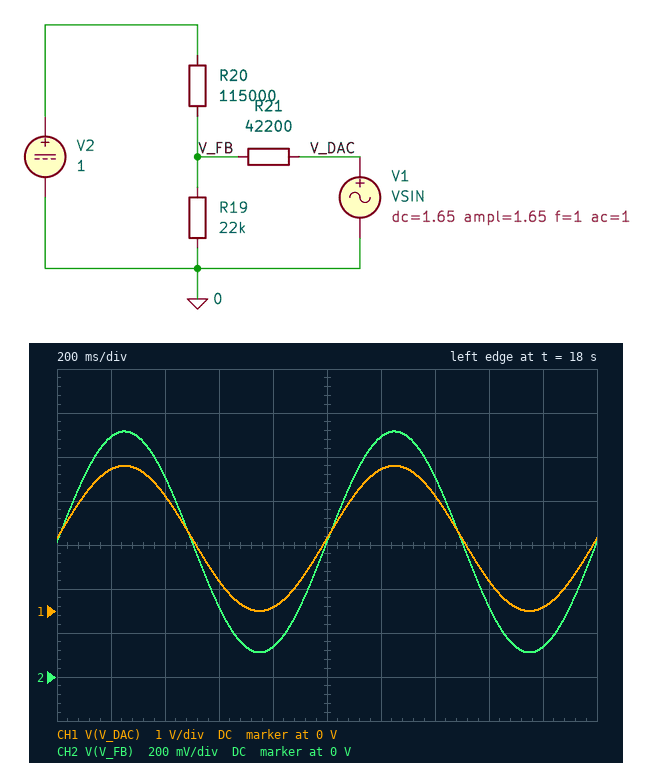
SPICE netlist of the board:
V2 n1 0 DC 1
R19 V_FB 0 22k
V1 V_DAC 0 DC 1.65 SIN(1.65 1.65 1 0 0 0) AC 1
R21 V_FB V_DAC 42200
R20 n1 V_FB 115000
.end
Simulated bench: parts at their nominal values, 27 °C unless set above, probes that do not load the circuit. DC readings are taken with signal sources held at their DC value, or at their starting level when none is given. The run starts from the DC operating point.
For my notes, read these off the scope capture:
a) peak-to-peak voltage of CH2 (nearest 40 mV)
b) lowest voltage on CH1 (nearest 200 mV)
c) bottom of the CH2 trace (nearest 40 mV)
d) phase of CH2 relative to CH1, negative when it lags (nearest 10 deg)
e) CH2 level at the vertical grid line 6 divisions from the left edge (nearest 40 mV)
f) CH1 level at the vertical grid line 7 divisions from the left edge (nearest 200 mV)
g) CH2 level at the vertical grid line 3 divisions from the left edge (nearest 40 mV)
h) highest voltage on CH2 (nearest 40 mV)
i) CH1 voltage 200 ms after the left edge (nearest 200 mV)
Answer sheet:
1.00 V
0 V
120 mV
0 deg
1.08 V
2.6 V
320 mV
1.12 V
3.2 V
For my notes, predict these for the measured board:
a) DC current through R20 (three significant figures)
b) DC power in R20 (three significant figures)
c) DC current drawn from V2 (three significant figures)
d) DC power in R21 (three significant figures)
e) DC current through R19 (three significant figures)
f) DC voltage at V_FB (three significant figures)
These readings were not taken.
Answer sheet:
3.36 µA
1.30 µW
3.36 µA
25.4 µW
27.9 µA
614 mV
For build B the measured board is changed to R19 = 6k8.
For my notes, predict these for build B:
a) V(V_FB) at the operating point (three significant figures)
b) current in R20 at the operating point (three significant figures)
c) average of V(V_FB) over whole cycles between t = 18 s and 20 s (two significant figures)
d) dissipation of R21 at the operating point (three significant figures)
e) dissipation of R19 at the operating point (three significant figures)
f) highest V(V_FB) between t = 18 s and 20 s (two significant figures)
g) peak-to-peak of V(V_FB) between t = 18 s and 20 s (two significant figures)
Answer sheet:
266 mV
6.38 µA
270 mV
45.4 µW
10.4 µW
480 mV
440 mV
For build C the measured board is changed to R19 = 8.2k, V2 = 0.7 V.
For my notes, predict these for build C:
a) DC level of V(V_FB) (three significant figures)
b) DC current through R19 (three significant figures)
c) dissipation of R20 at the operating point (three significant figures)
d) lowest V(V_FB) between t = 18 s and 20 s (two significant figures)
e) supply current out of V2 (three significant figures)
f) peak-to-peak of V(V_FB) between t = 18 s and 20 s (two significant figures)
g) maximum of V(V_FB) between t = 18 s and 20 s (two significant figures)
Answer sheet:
293 mV
35.7 µA
1.44 µW
39 mV
3.54 µA
510 mV
550 mV
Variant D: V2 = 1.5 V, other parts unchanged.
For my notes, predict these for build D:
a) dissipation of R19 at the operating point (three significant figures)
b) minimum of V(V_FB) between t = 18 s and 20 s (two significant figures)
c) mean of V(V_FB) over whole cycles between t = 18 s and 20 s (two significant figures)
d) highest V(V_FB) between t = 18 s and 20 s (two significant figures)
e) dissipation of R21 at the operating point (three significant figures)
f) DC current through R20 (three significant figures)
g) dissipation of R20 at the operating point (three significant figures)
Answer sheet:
20.4 µW
170 mV
670 mV
1.2 V
22.8 µW
7.22 µA
5.99 µW
